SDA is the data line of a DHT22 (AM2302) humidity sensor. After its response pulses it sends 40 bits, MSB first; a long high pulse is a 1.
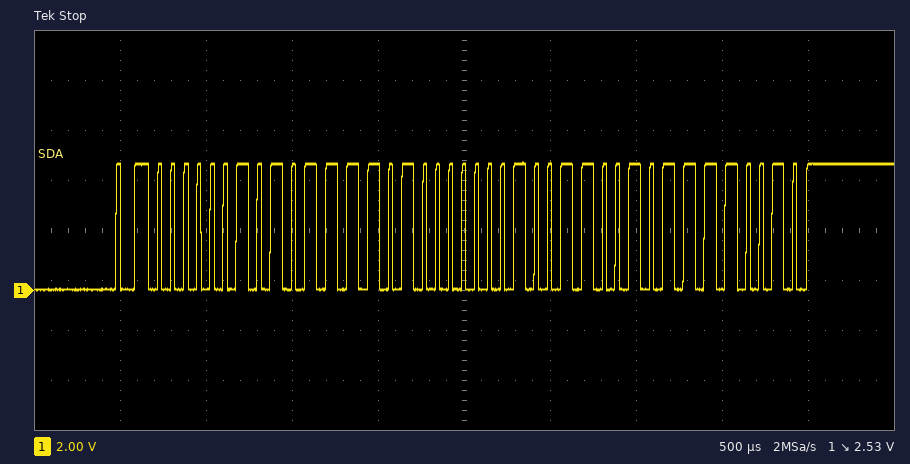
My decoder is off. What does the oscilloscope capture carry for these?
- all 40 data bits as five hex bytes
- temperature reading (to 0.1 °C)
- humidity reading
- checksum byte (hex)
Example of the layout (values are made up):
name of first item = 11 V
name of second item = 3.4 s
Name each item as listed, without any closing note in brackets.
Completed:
all 40 data bits as five hex bytes = 02 BD 01 32 F2
temperature reading = 30.6 °C
humidity reading = 70.1 %
checksum byte = 0xF2
